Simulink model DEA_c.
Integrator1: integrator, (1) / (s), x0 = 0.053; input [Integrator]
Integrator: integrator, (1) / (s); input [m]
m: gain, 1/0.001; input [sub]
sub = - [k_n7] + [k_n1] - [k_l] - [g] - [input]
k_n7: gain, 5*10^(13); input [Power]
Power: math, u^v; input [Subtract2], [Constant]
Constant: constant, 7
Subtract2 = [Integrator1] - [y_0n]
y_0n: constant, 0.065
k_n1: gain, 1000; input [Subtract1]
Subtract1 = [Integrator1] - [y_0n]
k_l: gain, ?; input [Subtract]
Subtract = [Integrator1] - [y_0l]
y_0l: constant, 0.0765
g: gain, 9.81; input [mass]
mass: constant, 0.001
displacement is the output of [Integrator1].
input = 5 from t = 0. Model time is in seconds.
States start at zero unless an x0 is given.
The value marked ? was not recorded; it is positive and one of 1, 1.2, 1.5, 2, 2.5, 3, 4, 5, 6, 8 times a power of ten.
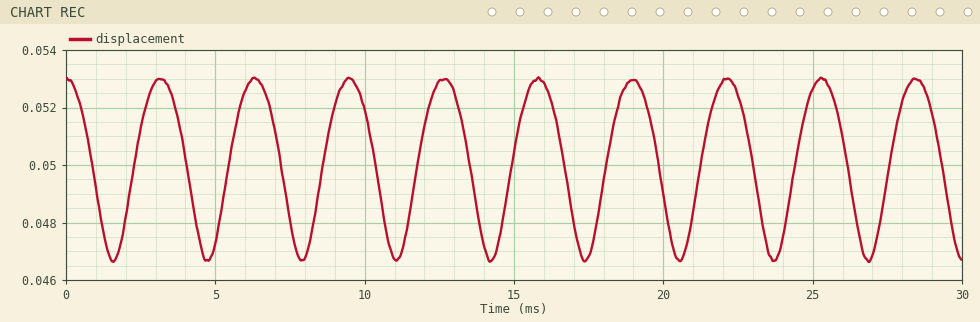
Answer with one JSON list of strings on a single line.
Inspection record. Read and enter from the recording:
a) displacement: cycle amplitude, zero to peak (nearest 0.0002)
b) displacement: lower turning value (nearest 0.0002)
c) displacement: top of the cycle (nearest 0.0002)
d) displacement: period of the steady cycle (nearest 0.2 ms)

["0.0032", "0.0466", "0.0530", "3.2 ms"]
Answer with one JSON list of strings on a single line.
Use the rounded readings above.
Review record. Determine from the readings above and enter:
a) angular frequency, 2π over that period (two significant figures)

["2.0 rad/ms"]
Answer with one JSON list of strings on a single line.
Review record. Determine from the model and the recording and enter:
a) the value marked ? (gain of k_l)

["300"]
